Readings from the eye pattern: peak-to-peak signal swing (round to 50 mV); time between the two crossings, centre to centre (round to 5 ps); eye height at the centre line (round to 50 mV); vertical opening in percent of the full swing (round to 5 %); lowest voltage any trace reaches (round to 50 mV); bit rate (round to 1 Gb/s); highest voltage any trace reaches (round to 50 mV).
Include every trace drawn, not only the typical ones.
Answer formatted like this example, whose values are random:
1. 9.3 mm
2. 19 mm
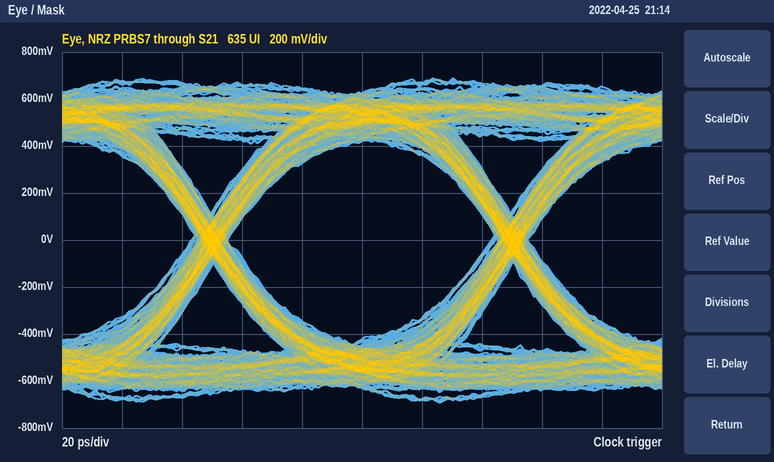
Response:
1. 1.40 V
2. 100 ps
3. 850 mV
4. 60 %
5. -700 mV
6. 10 Gb/s
7. 700 mV
